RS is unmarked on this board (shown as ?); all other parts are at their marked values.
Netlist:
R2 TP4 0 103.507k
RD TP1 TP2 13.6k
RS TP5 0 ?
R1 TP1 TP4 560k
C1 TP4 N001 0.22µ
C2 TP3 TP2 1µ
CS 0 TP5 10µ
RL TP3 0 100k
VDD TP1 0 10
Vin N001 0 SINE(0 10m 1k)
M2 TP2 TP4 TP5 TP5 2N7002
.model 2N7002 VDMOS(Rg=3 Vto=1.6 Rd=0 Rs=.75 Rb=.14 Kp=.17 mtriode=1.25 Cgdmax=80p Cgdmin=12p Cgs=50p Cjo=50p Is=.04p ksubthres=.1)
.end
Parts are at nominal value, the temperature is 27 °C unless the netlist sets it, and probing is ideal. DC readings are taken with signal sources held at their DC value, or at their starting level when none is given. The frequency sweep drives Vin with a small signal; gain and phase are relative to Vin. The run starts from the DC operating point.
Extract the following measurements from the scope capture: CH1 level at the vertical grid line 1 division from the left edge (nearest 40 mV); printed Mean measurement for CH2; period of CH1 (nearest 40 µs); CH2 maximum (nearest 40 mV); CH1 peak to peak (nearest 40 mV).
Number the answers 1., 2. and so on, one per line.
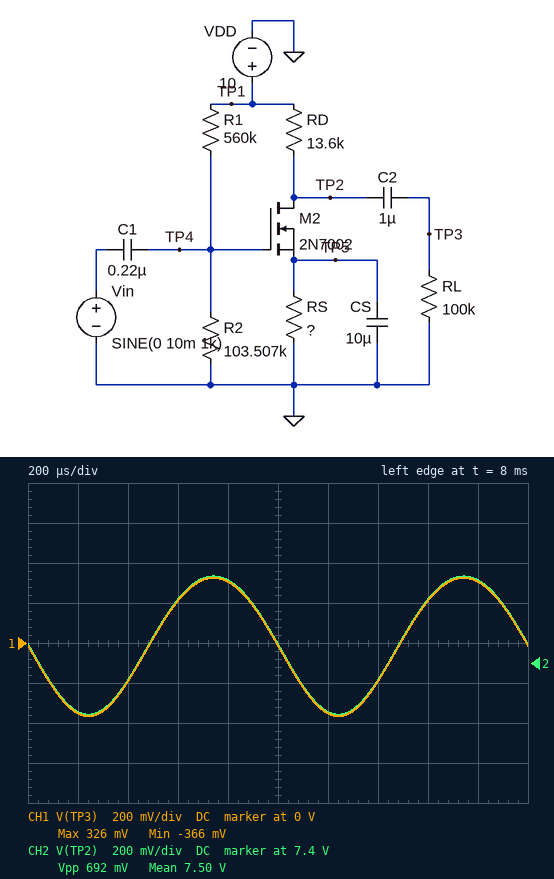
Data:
1. -360 mV
2. 7.50 V
3. 1.00 ms
4. 7.84 V
5. 680 mV
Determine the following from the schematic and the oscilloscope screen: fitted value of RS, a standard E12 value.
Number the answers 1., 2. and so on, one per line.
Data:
1. 68 Ω
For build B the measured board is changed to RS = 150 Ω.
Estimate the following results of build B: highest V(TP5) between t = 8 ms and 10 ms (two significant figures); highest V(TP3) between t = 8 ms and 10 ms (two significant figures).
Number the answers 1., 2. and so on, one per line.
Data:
1. 24 mV
2. 280 mV
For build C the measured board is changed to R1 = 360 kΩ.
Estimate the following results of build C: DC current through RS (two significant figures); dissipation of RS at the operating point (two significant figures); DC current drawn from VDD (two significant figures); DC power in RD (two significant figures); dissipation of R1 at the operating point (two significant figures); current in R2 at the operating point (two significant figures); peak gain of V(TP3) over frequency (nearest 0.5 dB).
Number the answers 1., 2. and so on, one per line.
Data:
1. 730 µA
2. 36 µW
3. 750 µA
4. 7.3 mW
5. 170 µW
6. 22 µA
7. -6.5 dB
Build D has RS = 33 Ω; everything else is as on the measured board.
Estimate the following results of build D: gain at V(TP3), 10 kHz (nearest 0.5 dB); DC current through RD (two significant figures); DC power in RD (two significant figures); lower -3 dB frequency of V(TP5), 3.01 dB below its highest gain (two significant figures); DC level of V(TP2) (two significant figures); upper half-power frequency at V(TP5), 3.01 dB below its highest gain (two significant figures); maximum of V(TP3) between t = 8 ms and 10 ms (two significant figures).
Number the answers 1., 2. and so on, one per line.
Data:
1. 31.5 dB
2. 200 µA
3. 550 µW
4. 8.0 Hz
5. 7.3 V
6. 550 Hz
7. 350 mV
